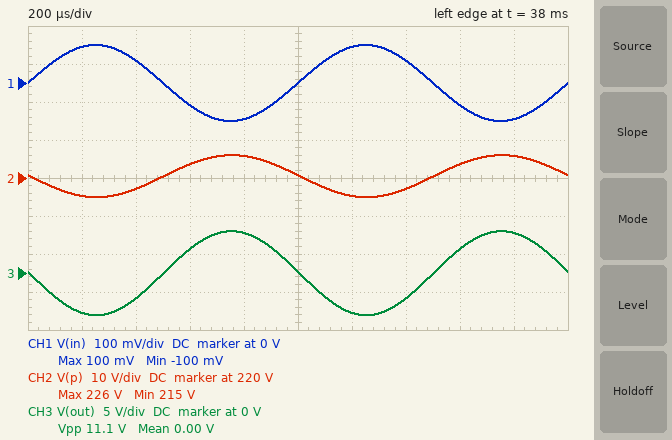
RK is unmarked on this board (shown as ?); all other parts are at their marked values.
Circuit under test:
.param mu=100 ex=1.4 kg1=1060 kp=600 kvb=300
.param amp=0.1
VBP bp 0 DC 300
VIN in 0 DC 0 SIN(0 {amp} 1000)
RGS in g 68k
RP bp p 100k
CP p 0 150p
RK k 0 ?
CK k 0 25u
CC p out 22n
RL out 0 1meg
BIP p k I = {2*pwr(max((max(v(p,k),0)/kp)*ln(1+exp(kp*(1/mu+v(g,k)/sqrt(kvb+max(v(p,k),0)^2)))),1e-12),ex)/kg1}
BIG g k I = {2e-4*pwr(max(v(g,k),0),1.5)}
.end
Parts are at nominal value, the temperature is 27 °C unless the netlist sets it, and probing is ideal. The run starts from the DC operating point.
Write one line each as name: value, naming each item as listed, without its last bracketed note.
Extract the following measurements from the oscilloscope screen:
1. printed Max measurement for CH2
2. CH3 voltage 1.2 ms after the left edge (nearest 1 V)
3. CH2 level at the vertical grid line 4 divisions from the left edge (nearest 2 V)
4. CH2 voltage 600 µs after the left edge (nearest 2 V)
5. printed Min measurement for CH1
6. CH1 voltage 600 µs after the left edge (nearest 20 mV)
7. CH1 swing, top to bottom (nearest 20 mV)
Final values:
printed Max measurement for CH2: 226 V
CH3 voltage 1.2 ms after the left edge: -5 V
CH2 level at the vertical grid line 4 divisions from the left edge: 226 V
CH2 voltage 600 µs after the left edge: 224 V
printed Min measurement for CH1: -100 mV
CH1 voltage 600 µs after the left edge: -60 mV
CH1 swing, top to bottom: 200 mV
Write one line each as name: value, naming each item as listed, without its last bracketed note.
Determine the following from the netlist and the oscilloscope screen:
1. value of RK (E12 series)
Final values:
value of RK: 2.2 kΩ
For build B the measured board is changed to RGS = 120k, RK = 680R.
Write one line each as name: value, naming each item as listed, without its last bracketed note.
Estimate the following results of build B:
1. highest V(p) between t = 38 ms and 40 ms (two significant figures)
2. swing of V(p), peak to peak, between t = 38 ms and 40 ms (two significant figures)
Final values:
highest V(p) between t = 38 ms and 40 ms: 170 V
swing of V(p), peak to peak, between t = 38 ms and 40 ms: 13 V
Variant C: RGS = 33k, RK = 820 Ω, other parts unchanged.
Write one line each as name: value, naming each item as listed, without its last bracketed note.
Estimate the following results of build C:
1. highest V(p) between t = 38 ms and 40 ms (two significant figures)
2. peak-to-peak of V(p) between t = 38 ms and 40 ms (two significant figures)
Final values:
highest V(p) between t = 38 ms and 40 ms: 180 V
peak-to-peak of V(p) between t = 38 ms and 40 ms: 13 V
